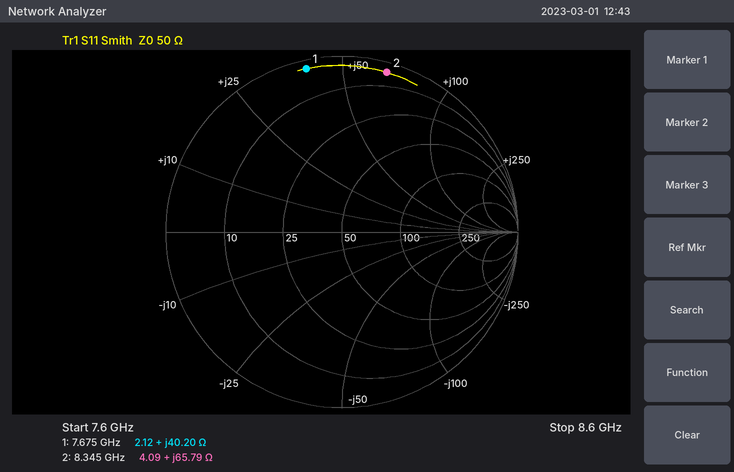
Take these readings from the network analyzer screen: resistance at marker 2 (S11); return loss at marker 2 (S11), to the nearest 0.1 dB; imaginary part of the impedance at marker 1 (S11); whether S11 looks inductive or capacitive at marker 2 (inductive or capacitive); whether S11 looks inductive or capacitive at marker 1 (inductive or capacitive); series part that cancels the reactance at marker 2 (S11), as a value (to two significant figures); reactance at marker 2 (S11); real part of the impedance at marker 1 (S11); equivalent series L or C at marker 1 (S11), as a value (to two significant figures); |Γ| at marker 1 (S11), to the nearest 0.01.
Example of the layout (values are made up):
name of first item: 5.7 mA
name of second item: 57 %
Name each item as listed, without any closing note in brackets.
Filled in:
resistance at marker 2: 4.09 Ω
return loss at marker 2 (S11), to the nearest 0.1 dB: 0.5 dB
imaginary part of the impedance at marker 1: +40.20 Ω
whether S11 looks inductive or capacitive at marker 2: inductive
whether S11 looks inductive or capacitive at marker 1: inductive
series part that cancels the reactance at marker 2 (S11), as a value: 290 fF
reactance at marker 2: +65.79 Ω
real part of the impedance at marker 1: 2.12 Ω
equivalent series L or C at marker 1 (S11), as a value: 830 pH
|Γ| at marker 1 (S11), to the nearest 0.01: 0.95
